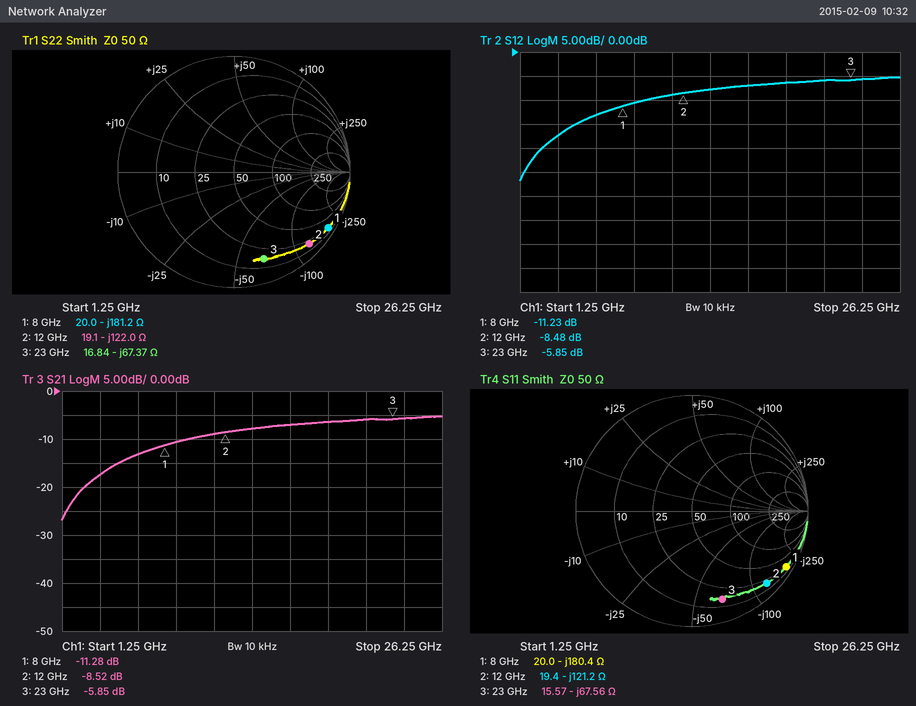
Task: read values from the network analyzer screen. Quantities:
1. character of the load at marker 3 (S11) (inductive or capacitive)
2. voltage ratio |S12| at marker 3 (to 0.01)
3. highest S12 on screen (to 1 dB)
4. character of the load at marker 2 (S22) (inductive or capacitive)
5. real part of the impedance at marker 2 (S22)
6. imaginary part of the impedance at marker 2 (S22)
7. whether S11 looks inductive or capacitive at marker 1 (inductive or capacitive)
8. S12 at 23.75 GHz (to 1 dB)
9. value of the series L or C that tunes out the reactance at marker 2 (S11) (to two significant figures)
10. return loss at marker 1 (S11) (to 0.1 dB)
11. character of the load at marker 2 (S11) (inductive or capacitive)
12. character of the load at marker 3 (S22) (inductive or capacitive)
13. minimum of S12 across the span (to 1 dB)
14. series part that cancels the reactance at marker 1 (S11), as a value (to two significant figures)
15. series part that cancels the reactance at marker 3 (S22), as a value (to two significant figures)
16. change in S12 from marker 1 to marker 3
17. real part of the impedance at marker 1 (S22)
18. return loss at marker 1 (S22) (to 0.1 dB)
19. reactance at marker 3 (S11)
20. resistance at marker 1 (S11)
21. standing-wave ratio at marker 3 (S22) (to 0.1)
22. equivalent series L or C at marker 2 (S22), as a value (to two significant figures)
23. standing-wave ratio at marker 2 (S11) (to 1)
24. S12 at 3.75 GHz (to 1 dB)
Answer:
capacitive
0.51
-5 dB
capacitive
19.1 Ω
-122.0 Ω
capacitive
-6 dB
1.6 nH
0.5 dB
capacitive
capacitive
-27 dB
3.6 nH
470 pH
5.38 dB
20.0 Ω
0.5 dB
-67.56 Ω
20.0 Ω
8.6
110 fF
18
-17 dB
